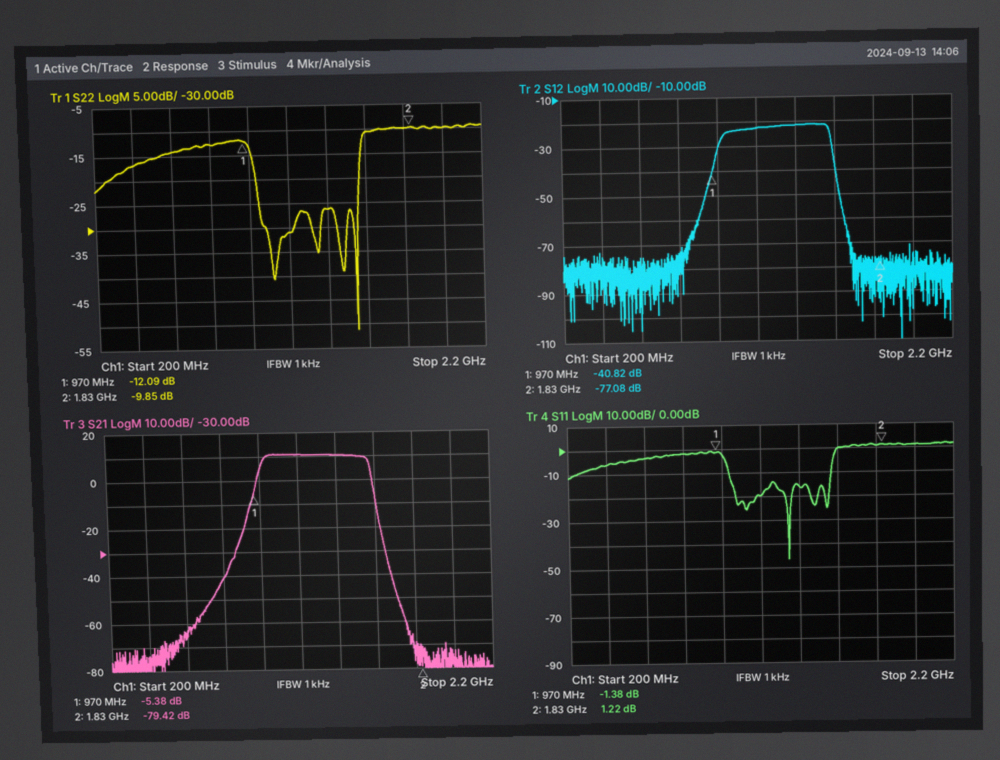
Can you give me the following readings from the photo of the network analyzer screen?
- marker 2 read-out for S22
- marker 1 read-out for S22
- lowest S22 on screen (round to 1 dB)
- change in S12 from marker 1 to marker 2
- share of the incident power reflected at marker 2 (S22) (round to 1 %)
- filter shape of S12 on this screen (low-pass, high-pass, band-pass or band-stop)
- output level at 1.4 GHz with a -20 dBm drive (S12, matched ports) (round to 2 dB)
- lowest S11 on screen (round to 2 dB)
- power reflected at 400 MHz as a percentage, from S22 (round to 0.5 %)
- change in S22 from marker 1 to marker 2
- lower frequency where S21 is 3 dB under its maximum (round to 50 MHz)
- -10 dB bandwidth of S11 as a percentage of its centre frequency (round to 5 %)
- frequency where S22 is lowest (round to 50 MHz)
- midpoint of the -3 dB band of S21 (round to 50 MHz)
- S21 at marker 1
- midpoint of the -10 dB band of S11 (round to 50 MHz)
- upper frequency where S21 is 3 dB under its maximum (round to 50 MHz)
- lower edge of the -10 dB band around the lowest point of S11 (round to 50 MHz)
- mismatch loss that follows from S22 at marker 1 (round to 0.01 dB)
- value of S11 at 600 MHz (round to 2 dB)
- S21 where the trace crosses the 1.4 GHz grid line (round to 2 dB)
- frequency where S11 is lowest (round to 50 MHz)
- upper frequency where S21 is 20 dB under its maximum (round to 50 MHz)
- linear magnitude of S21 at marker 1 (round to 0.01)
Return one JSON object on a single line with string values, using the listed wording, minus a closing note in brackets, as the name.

{"marker 2 read-out for S22": "-9.85 dB", "marker 1 read-out for S22": "-12.09 dB", "lowest S22 on screen": "-51 dB", "change in S12 from marker 1 to marker 2": "-36.26 dB", "share of the incident power reflected at marker 2 (S22)": "10 %", "filter shape of S12 on this screen": "band-pass", "output level at 1.4 GHz with a -20 dBm drive (S12, matched ports)": "-42 dBm", "lowest S11 on screen": "-46 dB", "power reflected at 400 MHz as a percentage, from S22": "2.0 %", "change in S22 from marker 1 to marker 2": "2.24 dB", "lower frequency where S21 is 3 dB under its maximum": "1.00 GHz", "-10 dB bandwidth of S11 as a percentage of its centre frequency": "40 %", "frequency where S22 is lowest": "1.55 GHz", "midpoint of the -3 dB band of S21": "1.30 GHz", "S21 at marker 1": "-5.38 dB", "midpoint of the -10 dB band of S11": "1.30 GHz", "upper frequency where S21 is 3 dB under its maximum": "1.55 GHz", "lower edge of the -10 dB band around the lowest point of S11": "1.05 GHz", "mismatch loss that follows from S22 at marker 1": "0.28 dB", "value of S11 at 600 MHz": "-4 dB", "S21 where the trace crosses the 1.4 GHz grid line": "10 dB", "frequency where S11 is lowest": "1.35 GHz", "upper frequency where S21 is 20 dB under its maximum": "1.60 GHz", "linear magnitude of S21 at marker 1": "0.54"}
